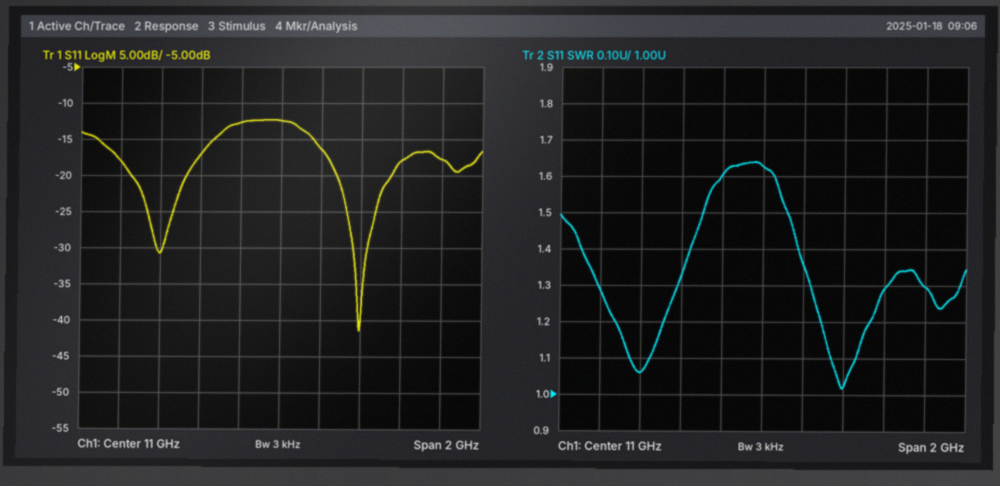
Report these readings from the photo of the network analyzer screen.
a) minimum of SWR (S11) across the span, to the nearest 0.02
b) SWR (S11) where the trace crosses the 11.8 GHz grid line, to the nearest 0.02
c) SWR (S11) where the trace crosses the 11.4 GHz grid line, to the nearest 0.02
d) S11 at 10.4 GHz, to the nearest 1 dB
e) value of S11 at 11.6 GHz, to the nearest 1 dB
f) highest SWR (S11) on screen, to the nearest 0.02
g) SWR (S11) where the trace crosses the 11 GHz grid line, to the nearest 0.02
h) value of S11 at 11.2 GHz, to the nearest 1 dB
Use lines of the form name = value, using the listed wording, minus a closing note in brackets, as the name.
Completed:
minimum of SWR (S11) across the span, to the nearest 0.02 = 1.02
SWR (S11) where the trace crosses the 11.8 GHz grid line, to the nearest 0.02 = 1.30
SWR (S11) where the trace crosses the 11.4 GHz grid line, to the nearest 0.02 = 1.02
S11 at 10.4 GHz, to the nearest 1 dB = -31 dB
value of S11 at 11.6 GHz, to the nearest 1 dB = -18 dB
highest SWR (S11) on screen, to the nearest 0.02 = 1.64
SWR (S11) where the trace crosses the 11 GHz grid line, to the nearest 0.02 = 1.62
value of S11 at 11.2 GHz, to the nearest 1 dB = -16 dB
